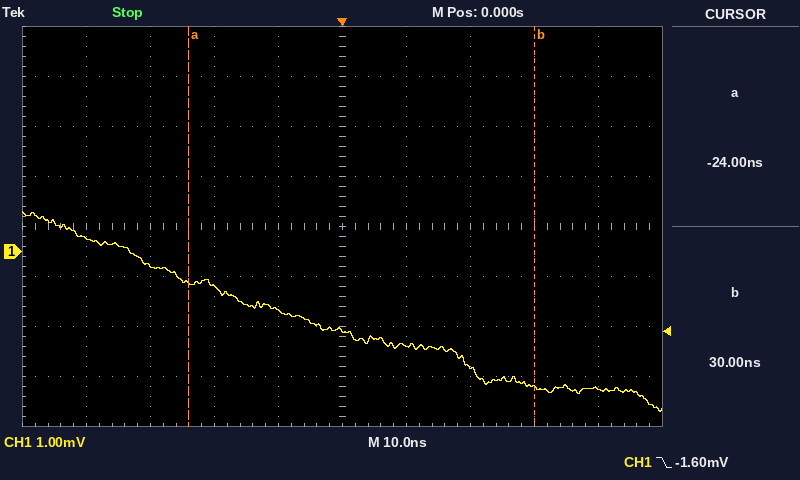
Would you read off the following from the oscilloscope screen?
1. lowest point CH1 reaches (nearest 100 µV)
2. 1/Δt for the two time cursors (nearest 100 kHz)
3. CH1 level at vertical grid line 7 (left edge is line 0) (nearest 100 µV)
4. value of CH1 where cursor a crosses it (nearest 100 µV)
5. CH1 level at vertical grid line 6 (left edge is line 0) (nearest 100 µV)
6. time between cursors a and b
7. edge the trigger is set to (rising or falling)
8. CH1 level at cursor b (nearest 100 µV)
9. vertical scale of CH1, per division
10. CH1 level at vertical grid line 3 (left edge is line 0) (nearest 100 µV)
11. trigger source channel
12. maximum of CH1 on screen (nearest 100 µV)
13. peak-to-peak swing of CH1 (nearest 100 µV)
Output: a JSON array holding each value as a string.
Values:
["-3.2 mV", "18.5 MHz", "-2.3 mV", "-600 µV", "-1.9 mV", "54 ns", "falling", "-2.7 mV", "1 mV", "-700 µV", "CH1", "800 µV", "4.0 mV"]
